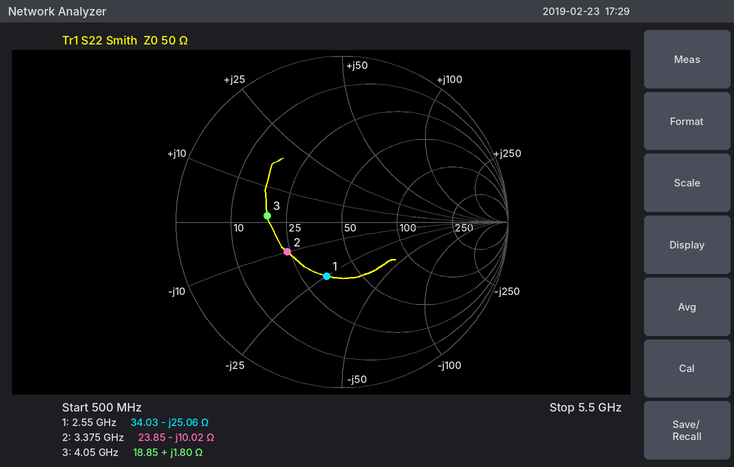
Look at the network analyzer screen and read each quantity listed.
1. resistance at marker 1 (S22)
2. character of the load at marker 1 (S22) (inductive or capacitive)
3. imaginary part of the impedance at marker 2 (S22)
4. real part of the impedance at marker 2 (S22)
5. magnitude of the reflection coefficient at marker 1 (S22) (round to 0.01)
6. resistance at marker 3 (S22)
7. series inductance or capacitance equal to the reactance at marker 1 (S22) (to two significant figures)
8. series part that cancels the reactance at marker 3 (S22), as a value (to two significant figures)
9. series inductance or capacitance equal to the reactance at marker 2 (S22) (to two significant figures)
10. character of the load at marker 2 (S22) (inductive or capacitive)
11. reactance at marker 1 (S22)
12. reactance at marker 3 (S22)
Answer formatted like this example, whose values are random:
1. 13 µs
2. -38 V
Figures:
1. 34.03 Ω
2. capacitive
3. -10.02 Ω
4. 23.85 Ω
5. 0.34
6. 18.85 Ω
7. 2.5 pF
8. 22 pF
9. 4.7 pF
10. capacitive
11. -25.06 Ω
12. +1.80 Ω
